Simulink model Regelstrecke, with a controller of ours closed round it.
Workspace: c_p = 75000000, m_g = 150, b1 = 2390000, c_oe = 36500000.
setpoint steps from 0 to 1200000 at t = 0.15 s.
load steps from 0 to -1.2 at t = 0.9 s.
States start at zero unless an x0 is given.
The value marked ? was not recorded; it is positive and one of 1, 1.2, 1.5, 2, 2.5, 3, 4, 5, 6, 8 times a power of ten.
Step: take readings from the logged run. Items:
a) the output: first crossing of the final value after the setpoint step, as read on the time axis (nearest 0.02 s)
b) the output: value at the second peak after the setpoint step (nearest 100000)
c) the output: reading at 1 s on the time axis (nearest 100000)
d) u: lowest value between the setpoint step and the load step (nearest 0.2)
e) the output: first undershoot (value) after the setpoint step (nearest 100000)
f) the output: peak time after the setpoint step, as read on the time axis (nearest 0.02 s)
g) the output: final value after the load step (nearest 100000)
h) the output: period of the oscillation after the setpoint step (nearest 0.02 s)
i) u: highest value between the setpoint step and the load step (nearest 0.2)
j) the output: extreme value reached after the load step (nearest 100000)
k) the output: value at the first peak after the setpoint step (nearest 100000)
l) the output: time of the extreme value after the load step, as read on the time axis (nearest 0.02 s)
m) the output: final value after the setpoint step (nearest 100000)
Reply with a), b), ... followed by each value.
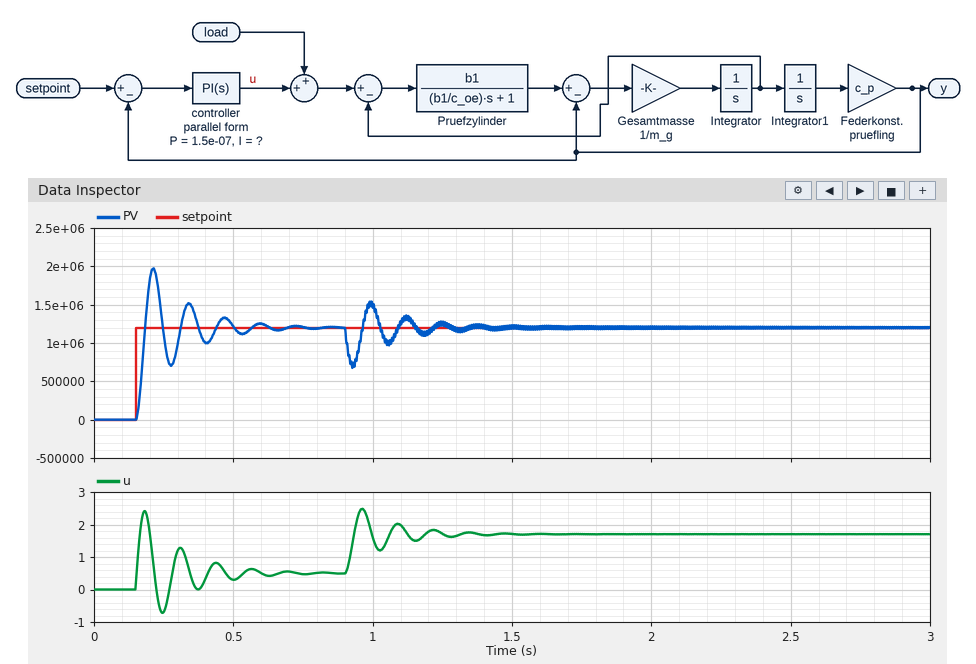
a) 0.18 s
b) 1500000
c) 1500000
d) -0.8
e) 700000
f) 0.22 s
g) 1200000
h) 0.12 s
i) 2.4
j) 700000
k) 2000000
l) 0.92 s
m) 1200000
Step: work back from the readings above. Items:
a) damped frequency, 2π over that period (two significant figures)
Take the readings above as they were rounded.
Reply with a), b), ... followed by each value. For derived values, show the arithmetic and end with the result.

a) 2π / 0.12 = 52 rad/s
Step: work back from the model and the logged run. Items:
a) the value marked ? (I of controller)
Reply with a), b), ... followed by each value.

a) 0.0001
